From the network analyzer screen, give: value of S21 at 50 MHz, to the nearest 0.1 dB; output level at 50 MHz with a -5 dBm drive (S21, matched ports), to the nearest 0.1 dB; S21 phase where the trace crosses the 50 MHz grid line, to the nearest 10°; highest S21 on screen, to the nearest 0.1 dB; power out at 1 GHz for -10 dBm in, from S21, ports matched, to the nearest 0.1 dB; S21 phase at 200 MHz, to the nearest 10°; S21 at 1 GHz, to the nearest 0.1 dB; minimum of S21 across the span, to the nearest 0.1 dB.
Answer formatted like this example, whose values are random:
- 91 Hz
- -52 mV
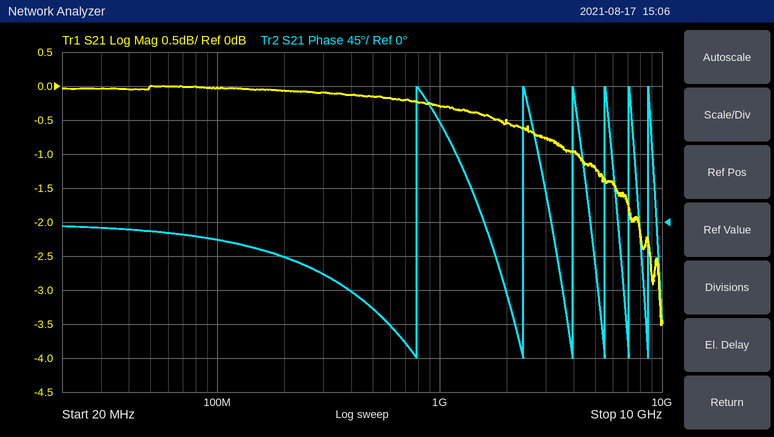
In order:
- 0.0 dB
- -5.0 dBm
- -10°
- 0.0 dB
- -10.3 dBm
- -50°
- -0.3 dB
- -3.5 dB
